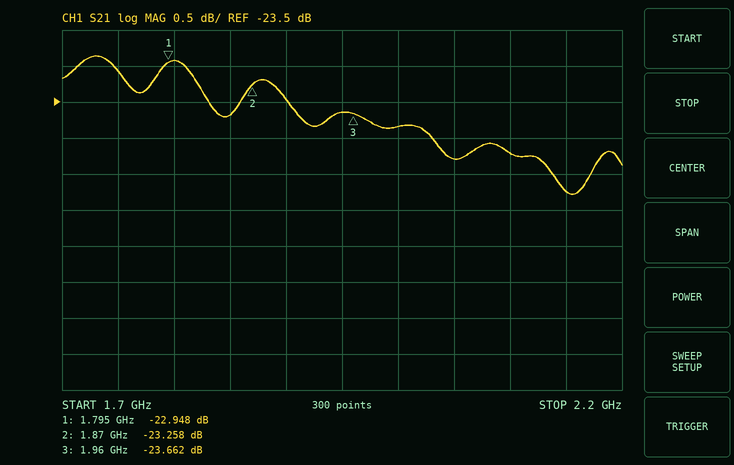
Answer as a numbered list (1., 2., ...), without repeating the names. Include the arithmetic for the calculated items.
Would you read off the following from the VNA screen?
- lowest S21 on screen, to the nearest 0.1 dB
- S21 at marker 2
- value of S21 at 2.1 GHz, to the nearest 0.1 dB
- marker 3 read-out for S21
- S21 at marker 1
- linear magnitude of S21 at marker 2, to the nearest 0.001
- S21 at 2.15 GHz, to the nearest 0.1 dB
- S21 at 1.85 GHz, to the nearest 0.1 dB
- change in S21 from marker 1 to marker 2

1. -24.8 dB
2. -23.258 dB
3. -24.2 dB
4. -23.662 dB
5. -22.948 dB
6. 10^(-23.258/20) ≈ 0.069
7. -24.7 dB
8. -23.7 dB
9. -23.258 − (-22.948) = -0.310 dB
